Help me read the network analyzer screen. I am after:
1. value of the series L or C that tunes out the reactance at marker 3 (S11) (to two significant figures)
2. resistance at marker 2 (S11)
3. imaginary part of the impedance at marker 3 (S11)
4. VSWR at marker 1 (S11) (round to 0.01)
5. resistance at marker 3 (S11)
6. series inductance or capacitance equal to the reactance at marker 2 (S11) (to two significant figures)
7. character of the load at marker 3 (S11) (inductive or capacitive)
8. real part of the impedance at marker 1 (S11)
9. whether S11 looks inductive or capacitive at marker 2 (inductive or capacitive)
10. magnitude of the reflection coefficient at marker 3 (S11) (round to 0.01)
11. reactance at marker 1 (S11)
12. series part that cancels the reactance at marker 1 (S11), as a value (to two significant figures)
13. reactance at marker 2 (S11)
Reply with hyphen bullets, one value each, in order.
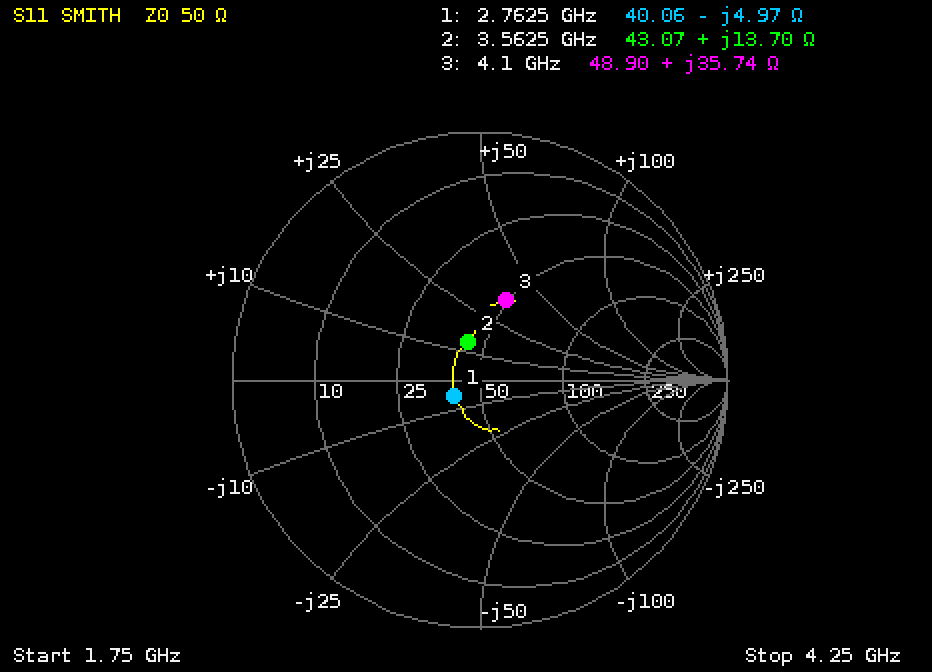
- 1.1 pF
- 43.07 Ω
- +35.74 Ω
- 1.28
- 48.90 Ω
- 610 pH
- inductive
- 40.06 Ω
- inductive
- 0.34
- -4.97 Ω
- 290 pH
- +13.70 Ω
